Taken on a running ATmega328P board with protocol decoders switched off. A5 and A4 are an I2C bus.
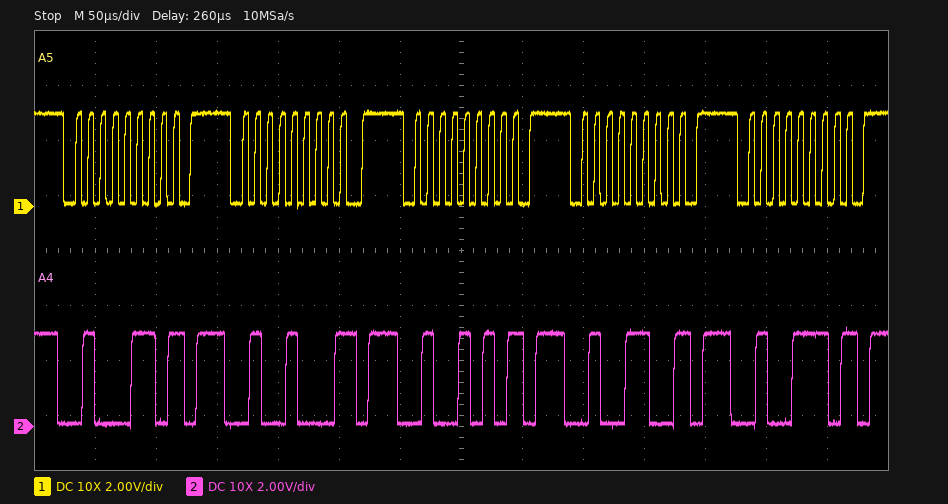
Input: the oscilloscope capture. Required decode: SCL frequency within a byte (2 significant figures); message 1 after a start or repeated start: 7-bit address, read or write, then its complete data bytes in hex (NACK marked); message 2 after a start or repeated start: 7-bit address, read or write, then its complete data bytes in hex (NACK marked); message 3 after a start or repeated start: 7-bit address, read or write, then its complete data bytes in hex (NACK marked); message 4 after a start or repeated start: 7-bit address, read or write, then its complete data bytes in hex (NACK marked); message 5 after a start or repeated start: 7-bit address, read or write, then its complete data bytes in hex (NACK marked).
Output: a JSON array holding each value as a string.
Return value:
["100 kHz", "0x23 write NACK", "0x24 write NACK", "0x25 write NACK", "0x26 write NACK", "0x27 write NACK"]
